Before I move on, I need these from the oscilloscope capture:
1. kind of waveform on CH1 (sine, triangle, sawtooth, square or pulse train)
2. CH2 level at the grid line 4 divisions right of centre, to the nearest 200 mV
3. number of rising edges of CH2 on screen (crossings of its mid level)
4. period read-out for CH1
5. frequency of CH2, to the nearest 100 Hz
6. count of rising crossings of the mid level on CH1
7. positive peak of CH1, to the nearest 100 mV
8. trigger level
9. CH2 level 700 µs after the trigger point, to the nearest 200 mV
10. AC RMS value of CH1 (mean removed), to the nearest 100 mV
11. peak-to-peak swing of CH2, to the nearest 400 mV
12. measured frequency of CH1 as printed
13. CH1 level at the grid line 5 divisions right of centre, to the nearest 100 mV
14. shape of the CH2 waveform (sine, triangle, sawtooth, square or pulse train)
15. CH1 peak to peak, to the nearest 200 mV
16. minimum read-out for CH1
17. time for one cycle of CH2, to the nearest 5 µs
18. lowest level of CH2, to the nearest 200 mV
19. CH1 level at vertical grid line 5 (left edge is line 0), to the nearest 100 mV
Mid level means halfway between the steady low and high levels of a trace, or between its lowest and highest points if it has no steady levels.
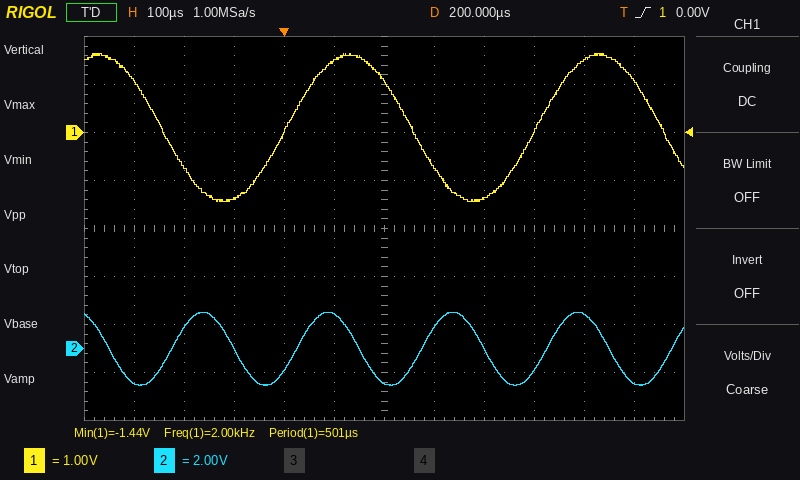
sine
1.4 V
5
501 µs
4.0 kHz
2
1.6 V
0.00 V
-1.4 V
1.1 V
3.2 V
2.00 kHz
1.1 V
sine
3.0 V
-1.44 V
250 µs
-1.6 V
1.5 V
